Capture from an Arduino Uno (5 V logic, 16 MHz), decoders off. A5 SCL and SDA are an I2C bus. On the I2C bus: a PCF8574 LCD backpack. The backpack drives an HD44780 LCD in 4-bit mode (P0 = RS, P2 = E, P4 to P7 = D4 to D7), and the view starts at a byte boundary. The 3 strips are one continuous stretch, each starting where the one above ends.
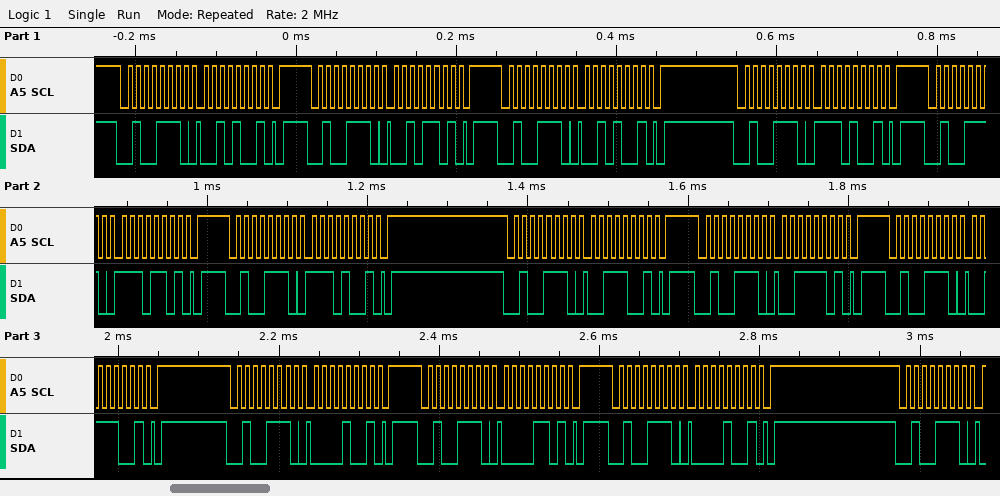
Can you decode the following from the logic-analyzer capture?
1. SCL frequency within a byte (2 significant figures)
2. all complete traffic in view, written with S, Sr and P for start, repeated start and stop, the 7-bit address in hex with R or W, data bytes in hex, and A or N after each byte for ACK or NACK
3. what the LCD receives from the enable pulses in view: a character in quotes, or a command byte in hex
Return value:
100 kHz
S 27W A 29 A P S 27W A 2D A P S 27W A 29 A P S 27W A E9 A P S 27W A ED A P S 27W A E9 A P S 27W A 39 A P S 27W A 3D A P S 27W A 39 A P S 27W A 09 A P S 27W A 0D A P S 27W A 09 A P S 27W A
'.' '0'
